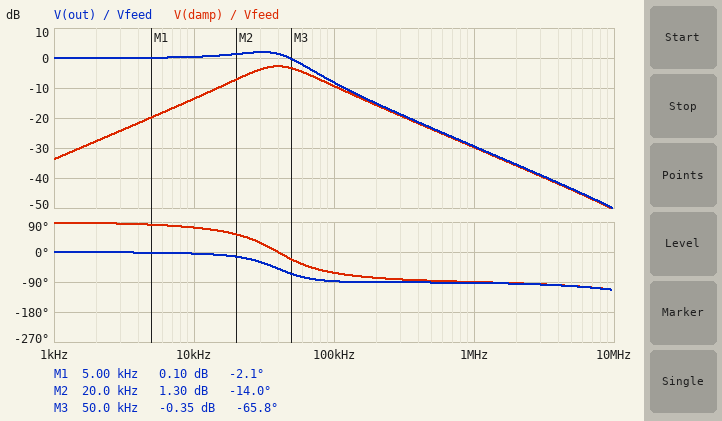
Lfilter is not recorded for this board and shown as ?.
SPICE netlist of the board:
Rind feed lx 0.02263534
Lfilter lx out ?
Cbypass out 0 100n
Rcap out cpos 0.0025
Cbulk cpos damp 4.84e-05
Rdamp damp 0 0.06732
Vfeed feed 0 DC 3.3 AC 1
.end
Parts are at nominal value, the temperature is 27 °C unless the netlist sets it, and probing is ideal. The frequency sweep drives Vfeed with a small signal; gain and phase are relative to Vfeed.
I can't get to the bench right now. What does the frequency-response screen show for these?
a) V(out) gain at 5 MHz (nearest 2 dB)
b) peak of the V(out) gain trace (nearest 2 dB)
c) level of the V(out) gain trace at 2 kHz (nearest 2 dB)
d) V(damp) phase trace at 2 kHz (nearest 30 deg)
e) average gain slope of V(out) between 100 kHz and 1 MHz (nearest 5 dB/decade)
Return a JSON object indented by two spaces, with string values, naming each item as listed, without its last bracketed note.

{
  "V(out) gain at 5 MHz": "-44 dB",
  "peak of the V(out) gain trace": "2 dB",
  "level of the V(out) gain trace at 2 kHz": "0 dB",
  "V(damp) phase trace at 2 kHz": "90 deg",
  "average gain slope of V(out) between 100 kHz and 1 MHz": "-20 dB/decade"
}
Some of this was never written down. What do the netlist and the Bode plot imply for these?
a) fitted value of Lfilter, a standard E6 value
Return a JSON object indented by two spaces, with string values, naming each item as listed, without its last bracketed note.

{
  "fitted value of Lfilter, a standard E6 value": "330 nH"
}
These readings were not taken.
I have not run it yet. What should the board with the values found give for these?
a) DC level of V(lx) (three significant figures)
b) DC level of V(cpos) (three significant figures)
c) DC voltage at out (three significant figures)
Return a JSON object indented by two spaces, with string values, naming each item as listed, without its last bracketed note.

{
  "DC level of V(lx)": "3.30 V",
  "DC level of V(cpos)": "3.30 V",
  "DC voltage at out": "3.30 V"
}
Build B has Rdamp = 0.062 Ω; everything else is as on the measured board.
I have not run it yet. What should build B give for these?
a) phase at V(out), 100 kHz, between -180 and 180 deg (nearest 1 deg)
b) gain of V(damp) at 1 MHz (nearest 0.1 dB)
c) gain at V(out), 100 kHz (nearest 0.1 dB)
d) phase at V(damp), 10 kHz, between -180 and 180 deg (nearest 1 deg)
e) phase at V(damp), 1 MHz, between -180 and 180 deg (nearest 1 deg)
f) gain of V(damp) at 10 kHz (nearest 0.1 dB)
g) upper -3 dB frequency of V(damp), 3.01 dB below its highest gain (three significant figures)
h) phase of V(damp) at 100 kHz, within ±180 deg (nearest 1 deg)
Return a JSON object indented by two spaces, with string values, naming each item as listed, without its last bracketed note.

{
  "phase at V(out), 100 kHz, between -180 and 180 deg": "-91 deg",
  "gain of V(damp) at 1 MHz": "-30.5 dB",
  "gain at V(out), 100 kHz": "-8.6 dB",
  "phase at V(damp), 10 kHz, between -180 and 180 deg": "74 deg",
  "phase at V(damp), 1 MHz, between -180 and 180 deg": "-90 deg",
  "gain of V(damp) at 10 kHz": "-14.3 dB",
  "upper -3 dB frequency of V(damp), 3.01 dB below its highest gain": "66.0 kHz",
  "phase of V(damp) at 100 kHz, within ±180 deg": "-64 deg"
}
